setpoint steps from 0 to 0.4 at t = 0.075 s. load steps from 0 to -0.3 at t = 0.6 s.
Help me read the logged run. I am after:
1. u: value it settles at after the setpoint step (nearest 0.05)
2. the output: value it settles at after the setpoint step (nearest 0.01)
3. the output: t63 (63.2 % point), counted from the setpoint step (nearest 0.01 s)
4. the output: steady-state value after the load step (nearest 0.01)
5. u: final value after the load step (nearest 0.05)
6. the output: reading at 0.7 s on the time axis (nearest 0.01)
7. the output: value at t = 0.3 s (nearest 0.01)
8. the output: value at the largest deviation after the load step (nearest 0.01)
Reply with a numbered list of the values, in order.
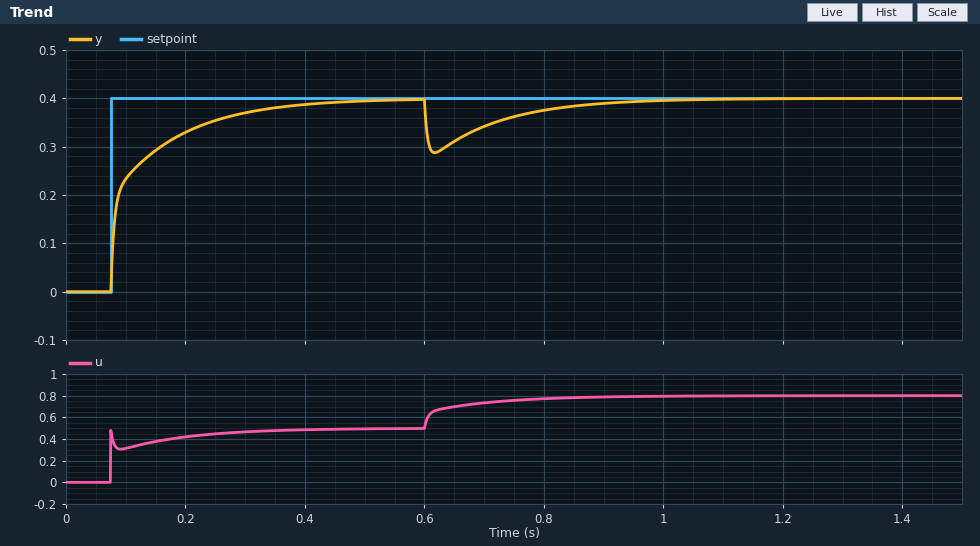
1. 0.50
2. 0.40
3. 0.04 s
4. 0.40
5. 0.80
6. 0.34
7. 0.37
8. 0.29
